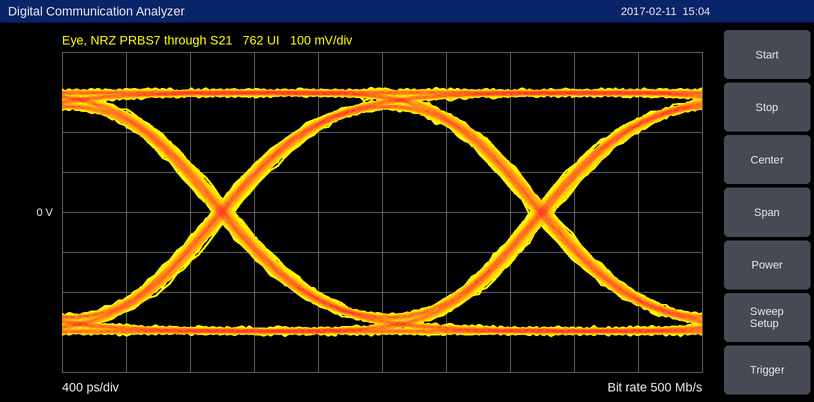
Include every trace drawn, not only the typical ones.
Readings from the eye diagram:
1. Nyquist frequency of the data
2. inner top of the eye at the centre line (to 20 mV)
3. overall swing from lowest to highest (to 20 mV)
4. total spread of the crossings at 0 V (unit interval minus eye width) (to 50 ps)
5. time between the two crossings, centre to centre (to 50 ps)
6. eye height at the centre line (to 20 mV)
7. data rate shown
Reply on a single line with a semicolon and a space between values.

250 MHz; 260 mV; 620 mV; 150 ps; 2.00 ns; 520 mV; 500 Mb/s
